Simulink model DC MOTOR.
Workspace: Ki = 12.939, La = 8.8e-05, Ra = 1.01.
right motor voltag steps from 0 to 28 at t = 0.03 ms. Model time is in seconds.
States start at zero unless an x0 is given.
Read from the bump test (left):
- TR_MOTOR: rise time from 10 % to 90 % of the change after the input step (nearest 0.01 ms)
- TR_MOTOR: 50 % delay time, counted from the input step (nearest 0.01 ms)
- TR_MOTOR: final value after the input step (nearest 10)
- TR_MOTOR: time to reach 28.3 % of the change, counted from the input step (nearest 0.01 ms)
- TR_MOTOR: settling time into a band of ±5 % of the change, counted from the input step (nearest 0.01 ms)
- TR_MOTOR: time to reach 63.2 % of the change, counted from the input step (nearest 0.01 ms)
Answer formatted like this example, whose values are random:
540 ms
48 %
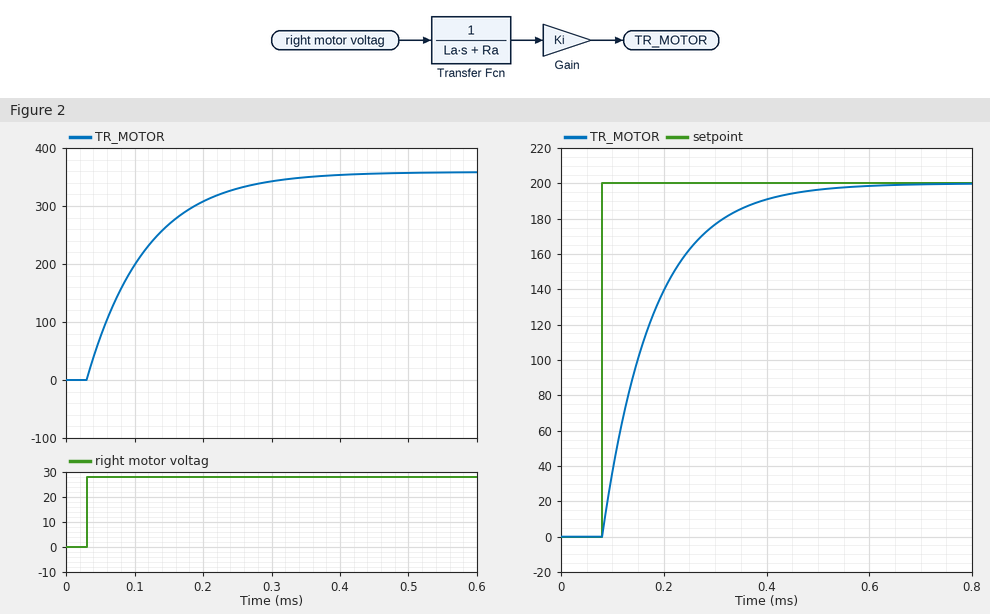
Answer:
0.19 ms
0.06 ms
360
0.03 ms
0.26 ms
0.09 ms
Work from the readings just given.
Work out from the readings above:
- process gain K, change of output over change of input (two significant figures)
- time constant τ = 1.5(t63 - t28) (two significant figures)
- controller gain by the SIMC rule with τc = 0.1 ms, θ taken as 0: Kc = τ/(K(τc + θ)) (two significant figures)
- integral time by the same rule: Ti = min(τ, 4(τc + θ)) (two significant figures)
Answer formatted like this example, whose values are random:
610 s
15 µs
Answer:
13
0.090 ms
0.069
0.090 ms
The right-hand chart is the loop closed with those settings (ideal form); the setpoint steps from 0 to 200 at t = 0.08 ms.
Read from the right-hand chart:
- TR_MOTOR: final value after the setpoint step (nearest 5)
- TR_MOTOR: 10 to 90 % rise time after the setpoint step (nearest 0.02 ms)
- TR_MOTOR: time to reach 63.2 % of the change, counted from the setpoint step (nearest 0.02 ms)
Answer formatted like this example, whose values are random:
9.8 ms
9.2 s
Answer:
200
0.22 ms
0.10 ms
